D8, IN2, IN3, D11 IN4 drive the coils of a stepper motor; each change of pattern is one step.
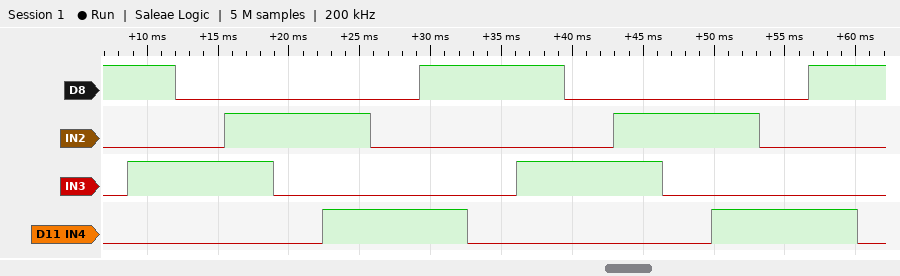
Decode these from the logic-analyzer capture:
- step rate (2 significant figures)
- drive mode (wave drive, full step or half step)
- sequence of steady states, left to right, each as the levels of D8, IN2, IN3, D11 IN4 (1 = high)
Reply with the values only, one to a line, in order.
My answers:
290 steps/s
half step
1000 1010 0010 0110 0100 0101 0001 1001 1000 1010 0010 0110 0100 0101 0001 1001 1000
